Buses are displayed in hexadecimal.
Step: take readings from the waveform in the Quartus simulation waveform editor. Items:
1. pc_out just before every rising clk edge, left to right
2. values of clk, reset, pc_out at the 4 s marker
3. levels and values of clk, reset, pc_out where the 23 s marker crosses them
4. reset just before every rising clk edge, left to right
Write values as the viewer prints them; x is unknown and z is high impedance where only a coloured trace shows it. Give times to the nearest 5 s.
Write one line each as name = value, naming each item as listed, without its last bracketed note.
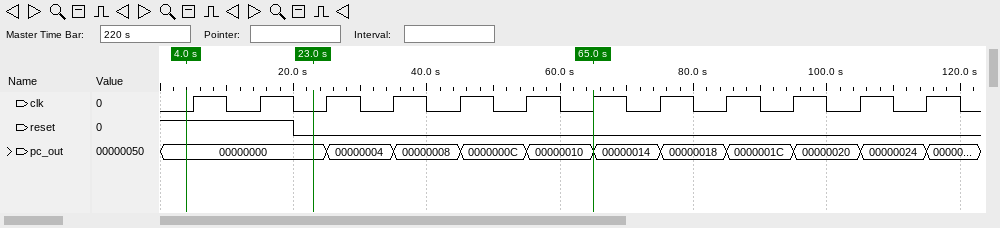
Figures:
pc_out just before every rising clk edge, left to right = 00000000, 00000000, 00000000, 00000004, 00000008, 0000000C, 00000010, 00000014, 00000018, 0000001C, 00000020, 00000024
values of clk, reset, pc_out at the 4 s marker = clk=0, reset=1, pc_out=00000000
levels and values of clk, reset, pc_out where the 23 s marker crosses them = clk=0, reset=0, pc_out=00000000
reset just before every rising clk edge, left to right = 1 1 0 0 0 0 0 0 0 0 0 0
